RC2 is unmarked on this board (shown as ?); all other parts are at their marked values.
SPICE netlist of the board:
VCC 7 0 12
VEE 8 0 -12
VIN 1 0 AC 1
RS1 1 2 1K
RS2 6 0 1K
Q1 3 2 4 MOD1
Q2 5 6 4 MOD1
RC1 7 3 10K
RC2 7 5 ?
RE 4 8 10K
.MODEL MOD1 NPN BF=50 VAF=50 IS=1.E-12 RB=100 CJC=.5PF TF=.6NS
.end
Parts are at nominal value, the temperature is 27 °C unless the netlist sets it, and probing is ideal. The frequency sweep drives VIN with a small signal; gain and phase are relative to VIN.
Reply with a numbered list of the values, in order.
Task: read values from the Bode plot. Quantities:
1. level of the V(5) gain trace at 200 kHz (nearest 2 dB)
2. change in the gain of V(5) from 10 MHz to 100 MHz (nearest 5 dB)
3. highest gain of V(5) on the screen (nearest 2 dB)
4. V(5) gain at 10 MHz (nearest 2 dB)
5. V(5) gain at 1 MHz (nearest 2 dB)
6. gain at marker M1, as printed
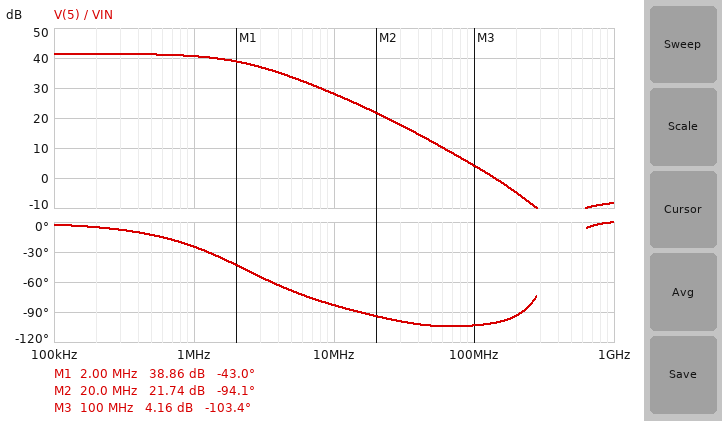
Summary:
1. 42 dB
2. -25 dB
3. 42 dB
4. 28 dB
5. 40 dB
6. 38.86 dB
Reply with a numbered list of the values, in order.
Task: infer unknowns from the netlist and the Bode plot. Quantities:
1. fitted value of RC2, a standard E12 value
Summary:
1. 18 kΩ
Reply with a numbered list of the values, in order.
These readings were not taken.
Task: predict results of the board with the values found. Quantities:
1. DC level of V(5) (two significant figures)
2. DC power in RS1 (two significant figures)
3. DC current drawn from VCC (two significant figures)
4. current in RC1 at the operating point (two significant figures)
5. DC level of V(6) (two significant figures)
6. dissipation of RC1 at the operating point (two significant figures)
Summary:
1. 2.2 V
2. 110 nW
3. 1.1 mA
4. 580 µA
5. -10 mV
6. 3.4 mW
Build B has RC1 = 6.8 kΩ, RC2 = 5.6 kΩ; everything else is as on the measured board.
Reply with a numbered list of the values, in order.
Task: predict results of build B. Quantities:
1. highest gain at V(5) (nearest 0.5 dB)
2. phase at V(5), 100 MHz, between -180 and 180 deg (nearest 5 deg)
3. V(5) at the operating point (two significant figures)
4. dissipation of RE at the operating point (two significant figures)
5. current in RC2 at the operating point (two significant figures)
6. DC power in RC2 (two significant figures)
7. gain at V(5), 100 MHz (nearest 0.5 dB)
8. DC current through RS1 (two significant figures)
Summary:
1. 32.0 dB
2. -95 deg
3. 8.8 V
4. 13 mW
5. 570 µA
6. 1.8 mW
7. 5.0 dB
8. 9.6 µA
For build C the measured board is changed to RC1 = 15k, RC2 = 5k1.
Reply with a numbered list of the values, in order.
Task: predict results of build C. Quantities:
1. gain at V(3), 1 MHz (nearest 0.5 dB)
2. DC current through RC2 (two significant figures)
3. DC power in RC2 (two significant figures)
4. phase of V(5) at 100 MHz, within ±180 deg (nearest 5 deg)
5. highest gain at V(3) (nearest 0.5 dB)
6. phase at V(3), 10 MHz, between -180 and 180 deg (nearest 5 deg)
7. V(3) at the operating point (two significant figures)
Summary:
1. 40.0 dB
2. 590 µA
3. 1.8 mW
4. -80 deg
5. 40.5 dB
6. 105 deg
7. 3.9 V
